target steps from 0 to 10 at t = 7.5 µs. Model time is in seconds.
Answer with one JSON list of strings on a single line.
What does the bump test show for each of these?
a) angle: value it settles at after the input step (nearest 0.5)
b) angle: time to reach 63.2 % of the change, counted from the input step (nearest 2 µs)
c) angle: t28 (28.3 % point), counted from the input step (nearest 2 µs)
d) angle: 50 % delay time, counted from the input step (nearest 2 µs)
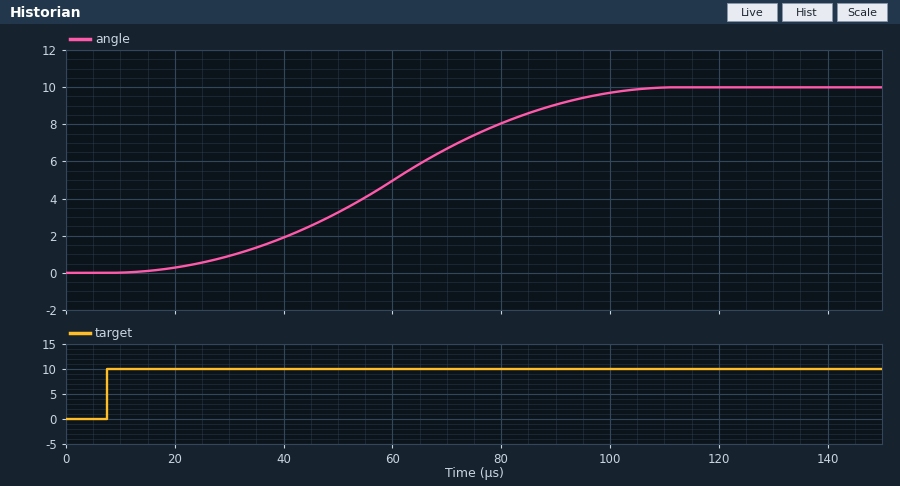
["10.0", "60 µs", "40 µs", "52 µs"]
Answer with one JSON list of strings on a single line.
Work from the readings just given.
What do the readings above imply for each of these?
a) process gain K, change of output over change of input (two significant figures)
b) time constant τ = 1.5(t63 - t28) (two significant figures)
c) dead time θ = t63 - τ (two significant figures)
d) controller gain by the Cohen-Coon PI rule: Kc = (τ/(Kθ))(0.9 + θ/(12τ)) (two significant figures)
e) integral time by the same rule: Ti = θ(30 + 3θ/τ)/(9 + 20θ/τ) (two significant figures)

["1.0", "30 µs", "30 µs", "0.98", "34 µs"]
